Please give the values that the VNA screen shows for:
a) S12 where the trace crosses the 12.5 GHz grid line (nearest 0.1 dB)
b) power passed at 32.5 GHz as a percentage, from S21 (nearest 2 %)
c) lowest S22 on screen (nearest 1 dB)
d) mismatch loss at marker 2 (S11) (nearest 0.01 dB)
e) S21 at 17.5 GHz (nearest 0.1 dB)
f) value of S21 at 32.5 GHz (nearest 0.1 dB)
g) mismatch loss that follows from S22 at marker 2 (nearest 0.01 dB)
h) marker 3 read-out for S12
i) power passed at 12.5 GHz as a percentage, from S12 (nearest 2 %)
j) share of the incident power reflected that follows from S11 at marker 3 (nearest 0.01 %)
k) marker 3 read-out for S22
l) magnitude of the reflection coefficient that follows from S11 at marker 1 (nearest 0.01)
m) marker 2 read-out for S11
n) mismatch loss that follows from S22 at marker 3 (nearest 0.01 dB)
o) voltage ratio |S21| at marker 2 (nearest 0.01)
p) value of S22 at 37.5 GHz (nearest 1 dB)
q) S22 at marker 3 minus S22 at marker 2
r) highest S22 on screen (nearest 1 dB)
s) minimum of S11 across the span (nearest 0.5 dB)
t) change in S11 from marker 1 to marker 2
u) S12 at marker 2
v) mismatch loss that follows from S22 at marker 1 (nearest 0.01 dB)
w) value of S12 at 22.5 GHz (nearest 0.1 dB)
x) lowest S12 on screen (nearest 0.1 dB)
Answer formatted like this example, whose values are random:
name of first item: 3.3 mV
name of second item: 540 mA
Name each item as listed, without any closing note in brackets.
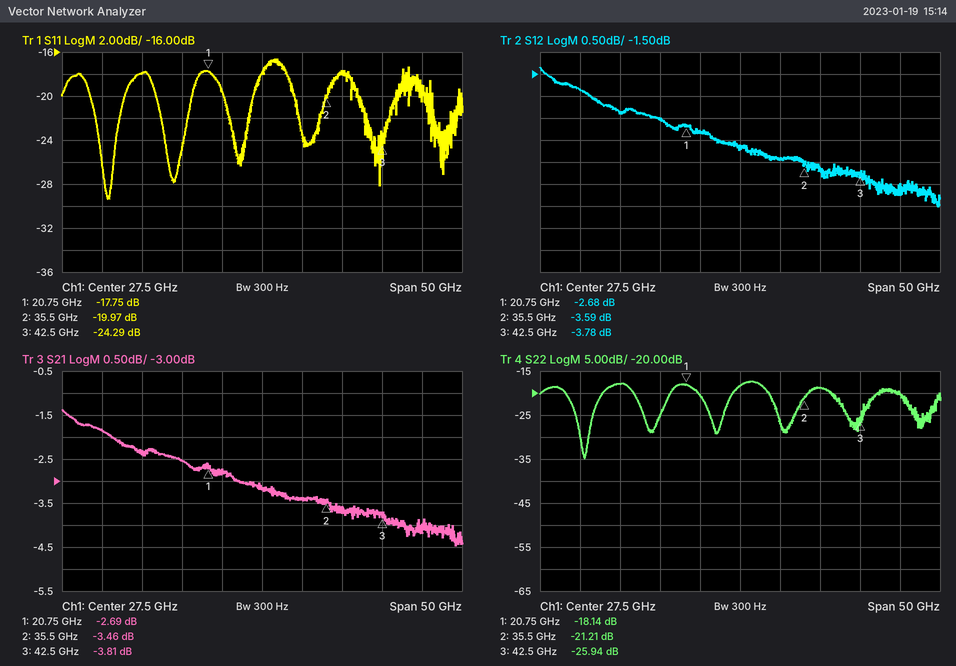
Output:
S12 where the trace crosses the 12.5 GHz grid line: -2.4 dB
power passed at 32.5 GHz as a percentage, from S21: 46 %
lowest S22 on screen: -35 dB
mismatch loss at marker 2 (S11): 0.04 dB
S21 at 17.5 GHz: -2.5 dB
value of S21 at 32.5 GHz: -3.4 dB
mismatch loss that follows from S22 at marker 2: 0.03 dB
marker 3 read-out for S12: -3.78 dB
power passed at 12.5 GHz as a percentage, from S12: 58 %
share of the incident power reflected that follows from S11 at marker 3: 0.37 %
marker 3 read-out for S22: -25.94 dB
magnitude of the reflection coefficient that follows from S11 at marker 1: 0.13
marker 2 read-out for S11: -19.97 dB
mismatch loss that follows from S22 at marker 3: 0.01 dB
voltage ratio |S21| at marker 2: 0.67
value of S22 at 37.5 GHz: -19 dB
S22 at marker 3 minus S22 at marker 2: -4.73 dB
highest S22 on screen: -17 dB
minimum of S11 across the span: -29.5 dB
change in S11 from marker 1 to marker 2: -2.22 dB
S12 at marker 2: -3.59 dB
mismatch loss that follows from S22 at marker 1: 0.07 dB
value of S12 at 22.5 GHz: -2.8 dB
lowest S12 on screen: -4.5 dB
